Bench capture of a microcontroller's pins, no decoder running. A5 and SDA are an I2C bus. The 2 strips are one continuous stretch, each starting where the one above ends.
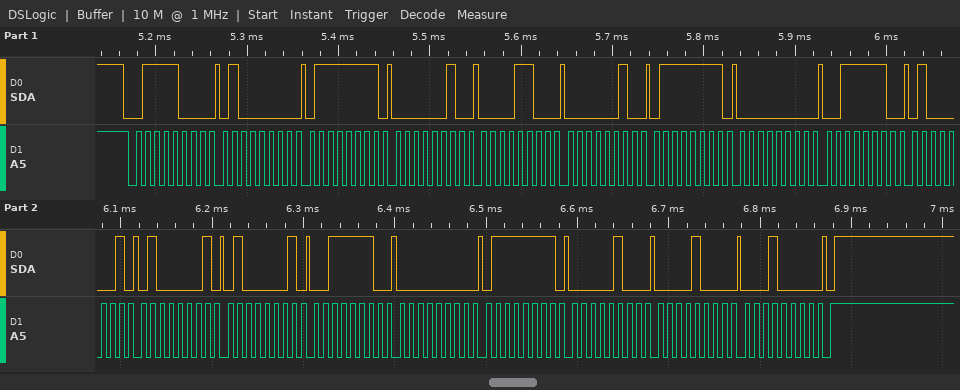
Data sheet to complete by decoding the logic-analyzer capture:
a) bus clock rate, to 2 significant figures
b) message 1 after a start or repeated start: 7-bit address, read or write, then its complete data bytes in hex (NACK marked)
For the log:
100 kHz
0x3C write: 40 7F 02 0C 02 7F 00 3E 41 41 41 3E 00 7F 04 08 10
